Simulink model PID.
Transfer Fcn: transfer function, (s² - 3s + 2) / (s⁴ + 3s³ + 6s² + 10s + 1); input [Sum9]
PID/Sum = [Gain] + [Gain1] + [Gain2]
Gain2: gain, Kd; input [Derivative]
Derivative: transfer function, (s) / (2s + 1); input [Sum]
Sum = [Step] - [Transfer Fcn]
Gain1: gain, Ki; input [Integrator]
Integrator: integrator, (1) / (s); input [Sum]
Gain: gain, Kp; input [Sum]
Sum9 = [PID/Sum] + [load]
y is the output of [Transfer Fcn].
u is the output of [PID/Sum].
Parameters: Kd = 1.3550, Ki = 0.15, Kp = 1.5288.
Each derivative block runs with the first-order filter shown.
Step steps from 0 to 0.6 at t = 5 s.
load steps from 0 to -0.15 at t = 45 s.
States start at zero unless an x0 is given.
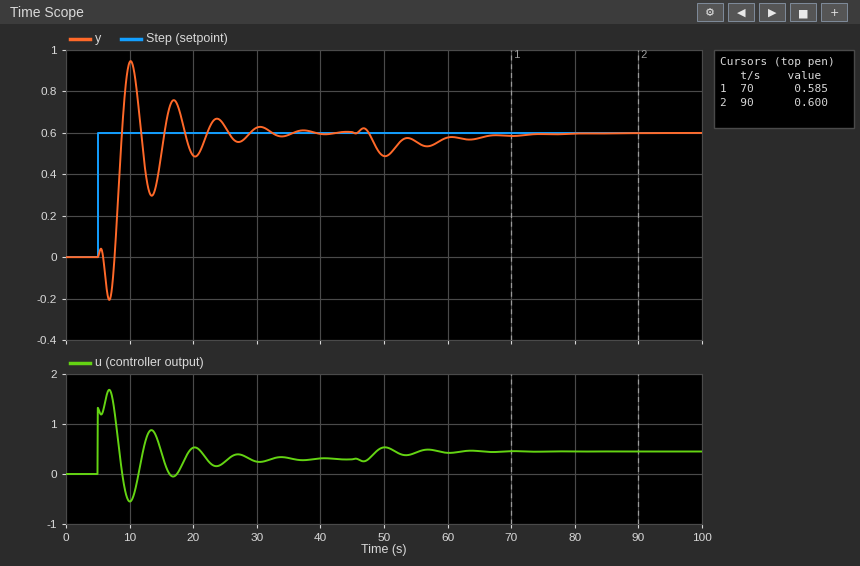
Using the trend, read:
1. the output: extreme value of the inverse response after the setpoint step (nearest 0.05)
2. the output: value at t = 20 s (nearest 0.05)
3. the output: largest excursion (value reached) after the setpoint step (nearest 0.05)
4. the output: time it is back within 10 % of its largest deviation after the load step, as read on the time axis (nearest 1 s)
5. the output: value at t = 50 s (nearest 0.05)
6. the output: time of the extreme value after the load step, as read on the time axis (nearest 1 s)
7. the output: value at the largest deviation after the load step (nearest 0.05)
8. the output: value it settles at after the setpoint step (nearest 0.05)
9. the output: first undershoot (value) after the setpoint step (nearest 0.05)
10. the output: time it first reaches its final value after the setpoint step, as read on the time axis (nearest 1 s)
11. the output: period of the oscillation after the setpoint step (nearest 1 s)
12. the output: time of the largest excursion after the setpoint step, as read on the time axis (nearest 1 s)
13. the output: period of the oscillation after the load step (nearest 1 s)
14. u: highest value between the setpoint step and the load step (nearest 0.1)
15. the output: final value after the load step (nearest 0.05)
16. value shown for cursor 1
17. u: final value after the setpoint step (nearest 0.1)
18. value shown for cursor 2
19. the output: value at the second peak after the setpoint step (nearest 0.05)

-0.20
0.50
0.95
72 s
0.50
50 s
0.50
0.60
0.30
9 s
7 s
10 s
7 s
1.7
0.60
0.585
0.3
0.600
0.75
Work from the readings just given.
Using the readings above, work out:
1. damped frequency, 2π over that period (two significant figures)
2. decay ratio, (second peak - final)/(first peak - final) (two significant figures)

0.90 rad/s
0.43
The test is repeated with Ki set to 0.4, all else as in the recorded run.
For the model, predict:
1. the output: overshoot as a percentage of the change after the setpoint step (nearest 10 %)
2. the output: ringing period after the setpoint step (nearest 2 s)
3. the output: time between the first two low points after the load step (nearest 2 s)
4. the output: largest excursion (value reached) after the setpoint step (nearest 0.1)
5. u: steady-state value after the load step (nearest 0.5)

90 %
8 s
8 s
1.2
0.5
